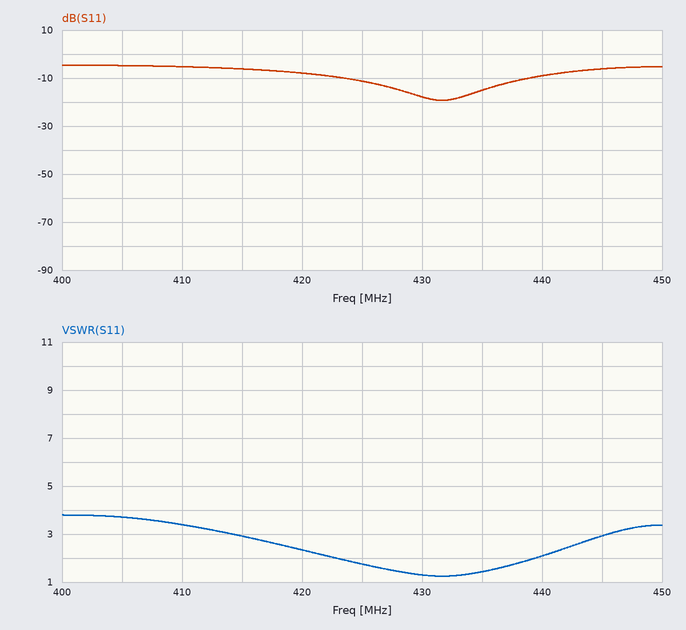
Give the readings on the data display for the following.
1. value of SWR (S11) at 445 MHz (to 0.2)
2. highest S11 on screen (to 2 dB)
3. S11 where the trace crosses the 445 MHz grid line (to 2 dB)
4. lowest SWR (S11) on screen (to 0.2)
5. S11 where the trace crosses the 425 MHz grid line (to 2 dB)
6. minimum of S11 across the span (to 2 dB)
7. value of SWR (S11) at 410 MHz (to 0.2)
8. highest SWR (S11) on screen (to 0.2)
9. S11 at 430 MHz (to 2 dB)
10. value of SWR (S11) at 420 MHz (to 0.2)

3.0
-4 dB
-6 dB
1.2
-12 dB
-20 dB
3.4
3.8
-18 dB
2.4
